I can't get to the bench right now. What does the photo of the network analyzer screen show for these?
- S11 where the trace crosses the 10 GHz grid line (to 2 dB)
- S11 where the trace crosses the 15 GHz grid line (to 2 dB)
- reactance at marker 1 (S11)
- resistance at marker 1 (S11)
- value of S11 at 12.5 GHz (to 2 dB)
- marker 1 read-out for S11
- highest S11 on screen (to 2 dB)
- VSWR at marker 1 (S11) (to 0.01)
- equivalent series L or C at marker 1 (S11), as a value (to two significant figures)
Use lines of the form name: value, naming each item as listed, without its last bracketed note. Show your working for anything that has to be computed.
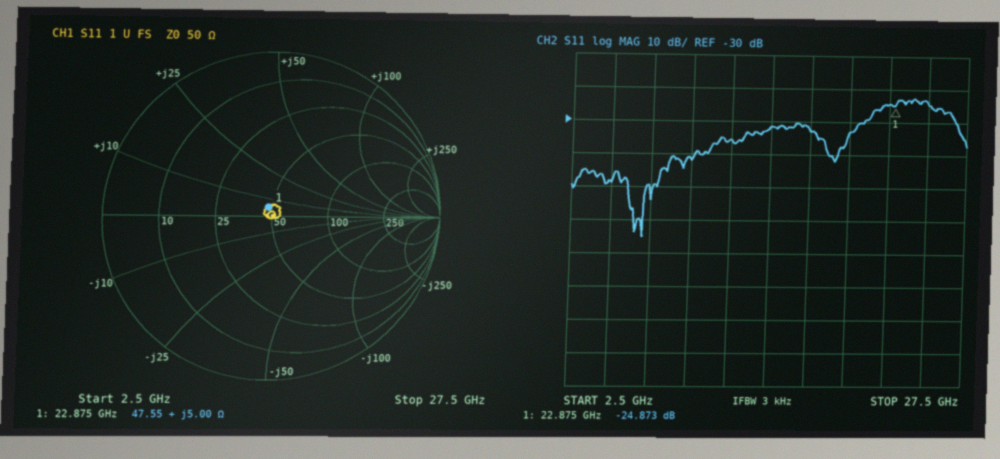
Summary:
S11 where the trace crosses the 10 GHz grid line: -42 dB
S11 where the trace crosses the 15 GHz grid line: -32 dB
reactance at marker 1: +5.00 Ω
resistance at marker 1: 47.55 Ω
value of S11 at 12.5 GHz: -36 dB
marker 1 read-out for S11: -24.873 dB
highest S11 on screen: -22 dB
VSWR at marker 1 (S11): 1.12
equivalent series L or C at marker 1 (S11), as a value: L = 5 Ω/(2π × 22.875 GHz) ≈ 35 pH
